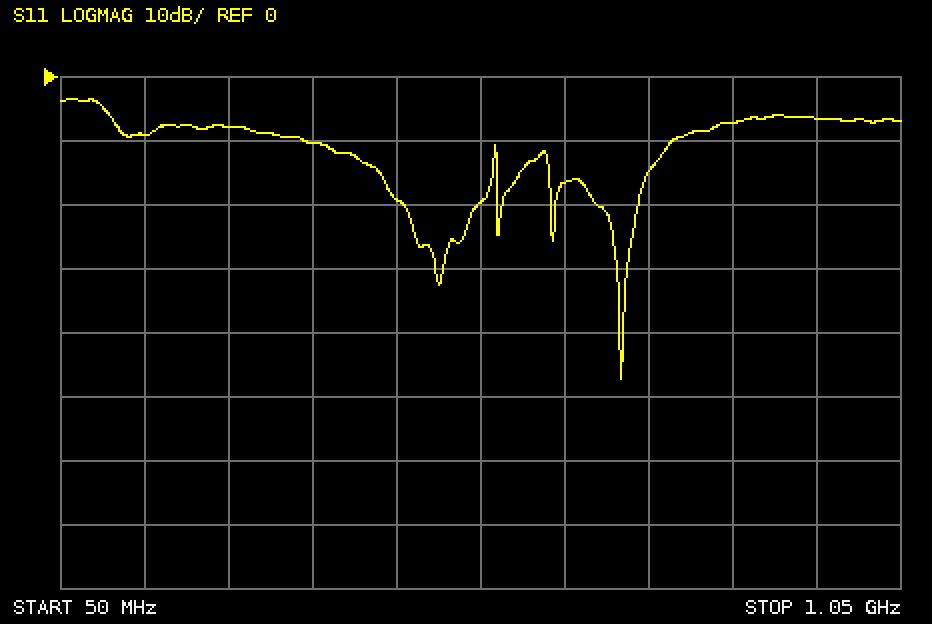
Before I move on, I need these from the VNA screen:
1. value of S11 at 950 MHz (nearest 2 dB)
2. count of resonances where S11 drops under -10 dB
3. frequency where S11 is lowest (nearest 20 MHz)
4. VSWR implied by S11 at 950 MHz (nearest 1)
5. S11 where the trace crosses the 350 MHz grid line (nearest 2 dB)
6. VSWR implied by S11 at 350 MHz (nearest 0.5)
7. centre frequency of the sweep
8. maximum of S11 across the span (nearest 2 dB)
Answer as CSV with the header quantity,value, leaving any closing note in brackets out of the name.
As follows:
quantity,value
value of S11 at 950 MHz,-6 dB
count of resonances where S11 drops under -10 dB,4
frequency where S11 is lowest,720 MHz
VSWR implied by S11 at 950 MHz,3
S11 where the trace crosses the 350 MHz grid line,-10 dB
VSWR implied by S11 at 350 MHz,2.0
centre frequency of the sweep,550 MHz
maximum of S11 across the span,-4 dB
